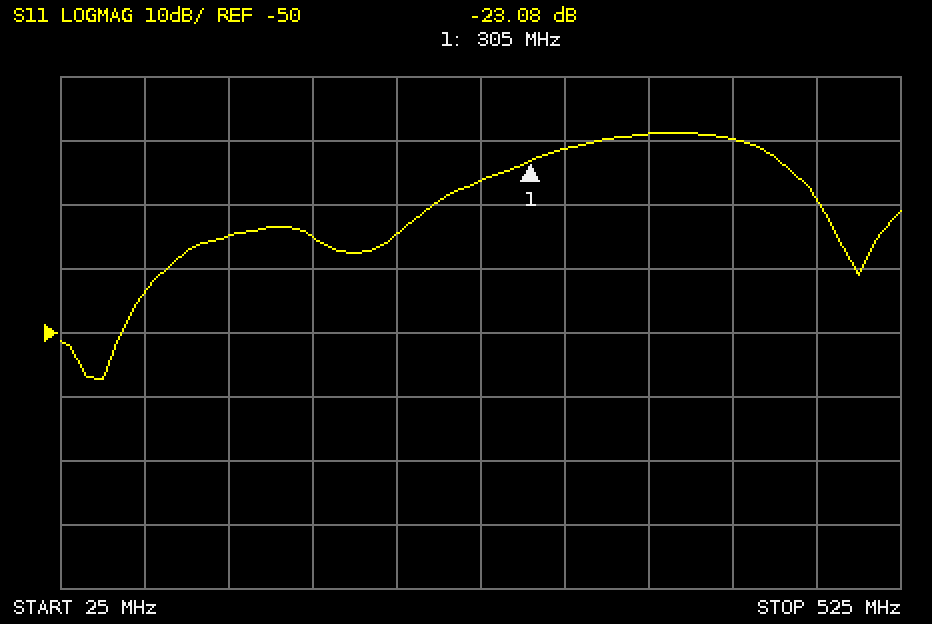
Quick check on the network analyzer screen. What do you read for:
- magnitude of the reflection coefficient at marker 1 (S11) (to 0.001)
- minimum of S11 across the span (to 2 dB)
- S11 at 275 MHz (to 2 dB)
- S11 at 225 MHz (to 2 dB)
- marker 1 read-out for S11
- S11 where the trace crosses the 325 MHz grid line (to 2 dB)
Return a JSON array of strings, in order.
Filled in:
["0.070", "-58 dB", "-26 dB", "-34 dB", "-23.08 dB", "-22 dB"]
